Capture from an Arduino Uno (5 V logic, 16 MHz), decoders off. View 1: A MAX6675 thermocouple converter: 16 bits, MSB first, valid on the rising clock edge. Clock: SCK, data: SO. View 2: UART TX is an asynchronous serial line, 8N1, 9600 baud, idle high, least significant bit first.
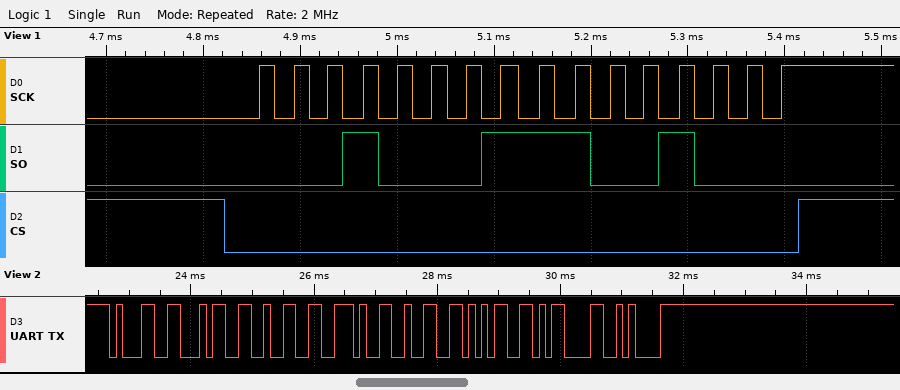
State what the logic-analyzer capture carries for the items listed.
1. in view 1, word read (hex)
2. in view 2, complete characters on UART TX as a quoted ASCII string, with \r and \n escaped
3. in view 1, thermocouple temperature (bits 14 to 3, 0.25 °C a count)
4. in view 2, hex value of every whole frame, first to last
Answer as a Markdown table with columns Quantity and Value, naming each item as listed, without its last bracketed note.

| Quantity | Value |
|---|---|
| in view 1, word read | 0x11C8 |
| in view 2, complete characters on UART TX as a quoted ASCII string, with \r and \n escaped | "142.25\r\n" |
| in view 1, thermocouple temperature | 142.25 °C |
| in view 2, hex value of every whole frame, first to last | 31 34 32 2E 32 35 0D 0A |
